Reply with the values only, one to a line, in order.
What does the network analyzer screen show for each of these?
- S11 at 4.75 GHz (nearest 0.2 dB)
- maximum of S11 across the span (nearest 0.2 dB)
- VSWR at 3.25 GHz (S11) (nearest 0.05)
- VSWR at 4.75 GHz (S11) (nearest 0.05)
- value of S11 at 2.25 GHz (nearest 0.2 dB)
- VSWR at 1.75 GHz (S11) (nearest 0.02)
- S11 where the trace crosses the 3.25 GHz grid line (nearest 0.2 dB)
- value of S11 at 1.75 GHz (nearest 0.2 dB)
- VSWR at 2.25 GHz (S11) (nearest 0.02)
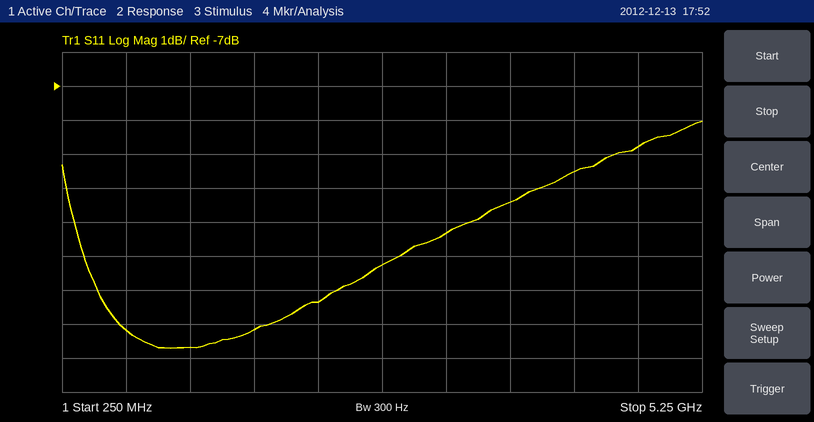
-8.8 dB
-8.0 dB
1.75
2.15
-13.4 dB
1.48
-11.4 dB
-14.2 dB
1.54
